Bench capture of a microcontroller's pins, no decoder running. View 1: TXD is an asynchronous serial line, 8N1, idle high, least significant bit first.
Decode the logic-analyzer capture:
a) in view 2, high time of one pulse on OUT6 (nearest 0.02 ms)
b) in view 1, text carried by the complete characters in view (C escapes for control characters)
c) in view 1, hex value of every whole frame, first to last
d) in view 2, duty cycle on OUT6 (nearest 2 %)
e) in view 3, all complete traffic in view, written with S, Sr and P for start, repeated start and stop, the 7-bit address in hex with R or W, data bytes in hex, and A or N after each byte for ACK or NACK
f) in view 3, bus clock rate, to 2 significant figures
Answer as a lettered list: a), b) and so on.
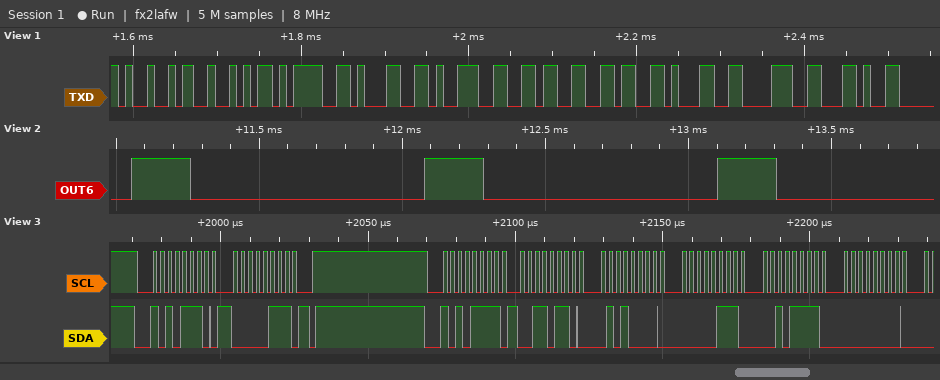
a) 0.20 ms
b) "IR=196618,"
c) 49 52 3D 31 39 36 36 31 38 2C
d) 20 %
e) S 57W A 07 A P S 57R A 36 A 50 A 07 A 2F A 00 A
f) 400 kHz
